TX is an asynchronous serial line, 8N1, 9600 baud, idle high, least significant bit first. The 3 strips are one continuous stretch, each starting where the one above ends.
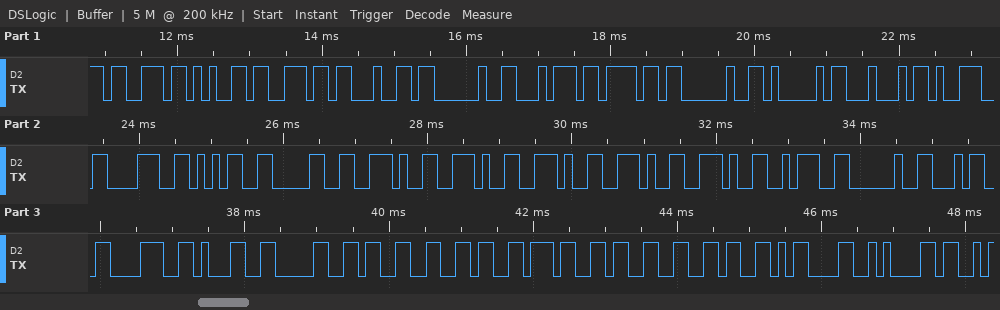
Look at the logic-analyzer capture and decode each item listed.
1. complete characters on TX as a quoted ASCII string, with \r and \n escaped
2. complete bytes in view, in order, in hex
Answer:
"send to AD9850.....: 481036736\r\n"
73 65 6E 64 20 74 6F 20 41 44 39 38 35 30 2E 2E 2E 2E 2E 3A 20 34 38 31 30 33 36 37 33 36 0D 0A
